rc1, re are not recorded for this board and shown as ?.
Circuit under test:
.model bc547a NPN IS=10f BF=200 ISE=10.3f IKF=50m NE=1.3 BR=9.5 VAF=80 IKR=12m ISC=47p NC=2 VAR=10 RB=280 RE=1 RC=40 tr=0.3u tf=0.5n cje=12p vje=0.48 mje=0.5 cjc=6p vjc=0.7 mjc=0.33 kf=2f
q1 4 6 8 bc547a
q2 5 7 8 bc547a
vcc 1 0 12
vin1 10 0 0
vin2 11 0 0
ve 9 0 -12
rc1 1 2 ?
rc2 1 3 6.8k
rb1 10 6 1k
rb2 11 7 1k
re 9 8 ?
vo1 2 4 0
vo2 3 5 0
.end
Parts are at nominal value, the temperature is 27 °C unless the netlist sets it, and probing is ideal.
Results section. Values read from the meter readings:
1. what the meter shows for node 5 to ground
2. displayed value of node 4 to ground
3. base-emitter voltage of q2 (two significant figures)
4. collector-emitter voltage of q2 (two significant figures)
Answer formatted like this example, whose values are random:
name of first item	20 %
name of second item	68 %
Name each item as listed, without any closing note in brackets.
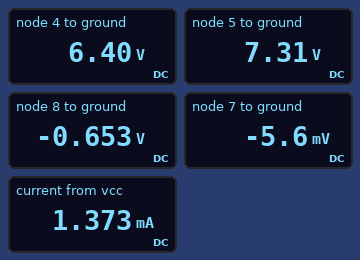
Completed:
what the meter shows for node 5 to ground	7.31 V
displayed value of node 4 to ground	6.40 V
base-emitter voltage of q2	650 mV
collector-emitter voltage of q2	8.0 V
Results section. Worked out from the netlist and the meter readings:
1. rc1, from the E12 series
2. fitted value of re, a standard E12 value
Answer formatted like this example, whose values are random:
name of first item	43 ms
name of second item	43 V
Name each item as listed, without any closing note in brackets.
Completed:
rc1, from the E12 series	8.2 kΩ
fitted value of re, a standard E12 value	8.2 kΩ
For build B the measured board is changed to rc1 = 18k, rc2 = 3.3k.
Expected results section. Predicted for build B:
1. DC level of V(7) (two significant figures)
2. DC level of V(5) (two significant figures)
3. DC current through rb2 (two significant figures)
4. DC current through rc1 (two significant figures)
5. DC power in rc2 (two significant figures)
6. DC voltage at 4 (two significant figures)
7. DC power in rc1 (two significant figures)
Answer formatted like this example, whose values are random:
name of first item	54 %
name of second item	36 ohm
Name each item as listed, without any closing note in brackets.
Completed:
DC level of V(7)	-5.7 mV
DC level of V(5)	9.6 V
DC current through rb2	5.7 µA
DC current through rc1	650 µA
DC power in rc2	1.7 mW
DC voltage at 4	350 mV
DC power in rc1	7.5 mW
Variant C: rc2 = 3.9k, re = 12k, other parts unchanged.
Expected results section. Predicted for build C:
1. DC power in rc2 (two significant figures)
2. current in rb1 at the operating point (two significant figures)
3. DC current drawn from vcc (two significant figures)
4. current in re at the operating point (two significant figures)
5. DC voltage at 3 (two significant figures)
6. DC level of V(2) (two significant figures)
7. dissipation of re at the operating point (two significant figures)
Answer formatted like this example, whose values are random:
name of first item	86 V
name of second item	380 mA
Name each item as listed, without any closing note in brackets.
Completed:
DC power in rc2	880 µW
current in rb1 at the operating point	3.9 µA
DC current drawn from vcc	940 µA
current in re at the operating point	950 µA
DC voltage at 3	10 V
DC level of V(2)	8.2 V
dissipation of re at the operating point	11 mW
